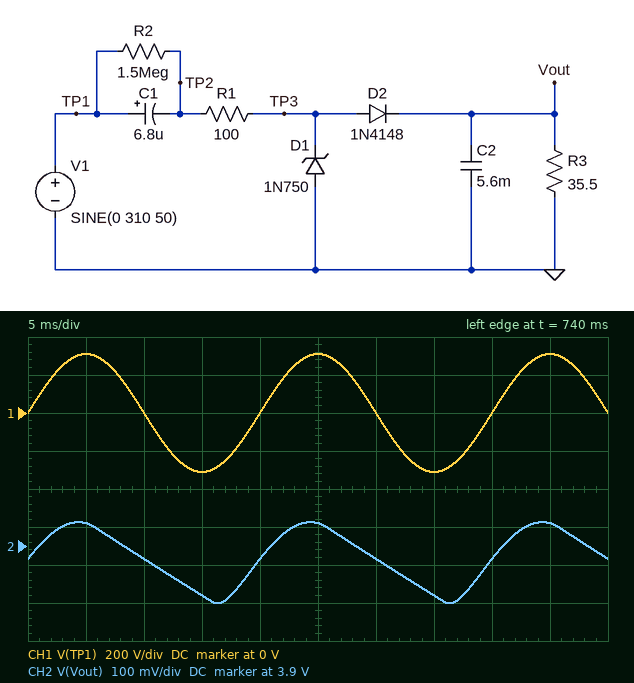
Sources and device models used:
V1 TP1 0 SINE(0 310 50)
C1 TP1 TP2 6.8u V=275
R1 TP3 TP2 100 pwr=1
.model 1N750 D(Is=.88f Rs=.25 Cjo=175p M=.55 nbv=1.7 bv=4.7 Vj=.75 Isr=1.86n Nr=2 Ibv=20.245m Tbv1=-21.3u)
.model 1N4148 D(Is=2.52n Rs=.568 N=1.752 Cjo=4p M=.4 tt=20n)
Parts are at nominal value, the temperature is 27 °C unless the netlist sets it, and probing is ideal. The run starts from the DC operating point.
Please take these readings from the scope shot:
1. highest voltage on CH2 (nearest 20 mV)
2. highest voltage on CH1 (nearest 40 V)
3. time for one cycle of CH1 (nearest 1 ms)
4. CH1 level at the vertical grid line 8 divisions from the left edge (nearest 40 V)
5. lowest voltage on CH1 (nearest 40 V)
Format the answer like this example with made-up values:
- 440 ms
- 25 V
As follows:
- 3.96 V
- 320 V
- 20 ms
- 0 V
- -320 V
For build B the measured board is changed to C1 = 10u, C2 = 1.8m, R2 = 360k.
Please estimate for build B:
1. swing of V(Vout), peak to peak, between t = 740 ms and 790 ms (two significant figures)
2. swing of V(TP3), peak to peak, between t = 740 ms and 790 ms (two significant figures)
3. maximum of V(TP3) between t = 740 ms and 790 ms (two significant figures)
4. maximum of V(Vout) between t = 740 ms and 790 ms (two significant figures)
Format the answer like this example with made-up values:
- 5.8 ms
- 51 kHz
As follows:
- 690 mV
- 6.2 V
- 5.0 V
- 4.1 V
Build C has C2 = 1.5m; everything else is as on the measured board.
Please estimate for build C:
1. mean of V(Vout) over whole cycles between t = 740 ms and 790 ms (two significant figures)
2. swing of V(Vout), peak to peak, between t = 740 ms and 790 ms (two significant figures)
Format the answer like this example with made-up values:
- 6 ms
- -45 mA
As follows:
- 3.7 V
- 790 mV
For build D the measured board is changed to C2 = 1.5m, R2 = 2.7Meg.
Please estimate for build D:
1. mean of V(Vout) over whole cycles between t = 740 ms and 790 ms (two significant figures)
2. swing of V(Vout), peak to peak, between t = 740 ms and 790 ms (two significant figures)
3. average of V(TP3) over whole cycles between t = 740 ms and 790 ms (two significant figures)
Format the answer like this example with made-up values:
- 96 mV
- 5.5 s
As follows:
- 3.7 V
- 790 mV
- 1.9 V
